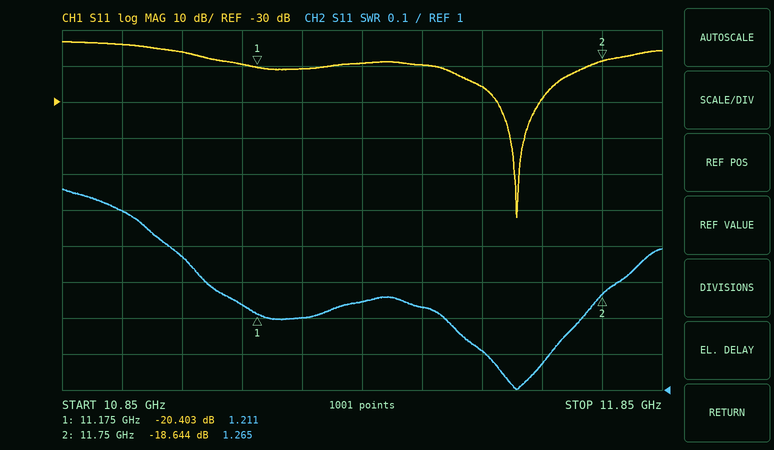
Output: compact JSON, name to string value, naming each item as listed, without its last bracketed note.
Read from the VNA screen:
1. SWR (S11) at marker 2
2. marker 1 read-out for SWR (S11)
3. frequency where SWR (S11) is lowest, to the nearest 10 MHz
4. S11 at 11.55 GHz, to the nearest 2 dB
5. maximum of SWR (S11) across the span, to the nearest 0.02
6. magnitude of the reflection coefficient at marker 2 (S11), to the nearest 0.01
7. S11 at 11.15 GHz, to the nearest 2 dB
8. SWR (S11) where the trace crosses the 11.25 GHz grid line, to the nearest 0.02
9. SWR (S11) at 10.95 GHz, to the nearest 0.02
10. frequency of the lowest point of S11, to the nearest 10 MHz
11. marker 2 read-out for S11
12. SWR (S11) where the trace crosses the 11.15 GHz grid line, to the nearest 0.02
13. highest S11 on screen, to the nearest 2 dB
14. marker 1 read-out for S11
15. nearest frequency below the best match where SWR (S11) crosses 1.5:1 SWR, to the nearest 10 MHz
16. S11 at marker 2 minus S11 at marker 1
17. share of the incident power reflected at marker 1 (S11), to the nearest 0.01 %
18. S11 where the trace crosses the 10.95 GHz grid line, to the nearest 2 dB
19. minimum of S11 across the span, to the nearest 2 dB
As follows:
{"SWR (S11) at marker 2": "1.265", "marker 1 read-out for SWR": "1.211", "frequency where SWR (S11) is lowest, to the nearest 10 MHz": "11.61 GHz", "S11 at 11.55 GHz, to the nearest 2 dB": "-26 dB", "maximum of SWR (S11) across the span, to the nearest 0.02": "1.56", "magnitude of the reflection coefficient at marker 2 (S11), to the nearest 0.01": "0.12", "S11 at 11.15 GHz, to the nearest 2 dB": "-20 dB", "SWR (S11) where the trace crosses the 11.25 GHz grid line, to the nearest 0.02": "1.20", "SWR (S11) at 10.95 GHz, to the nearest 0.02": "1.50", "frequency of the lowest point of S11, to the nearest 10 MHz": "11.61 GHz", "marker 2 read-out for S11": "-18.644 dB", "SWR (S11) where the trace crosses the 11.15 GHz grid line, to the nearest 0.02": "1.24", "highest S11 on screen, to the nearest 2 dB": "-14 dB", "marker 1 read-out for S11": "-20.403 dB", "nearest frequency below the best match where SWR (S11) crosses 1.5:1 SWR, to the nearest 10 MHz": "10.95 GHz", "S11 at marker 2 minus S11 at marker 1": "1.759 dB", "share of the incident power reflected at marker 1 (S11), to the nearest 0.01 %": "0.91 %", "S11 where the trace crosses the 10.95 GHz grid line, to the nearest 2 dB": "-14 dB", "minimum of S11 across the span, to the nearest 2 dB": "-62 dB"}
